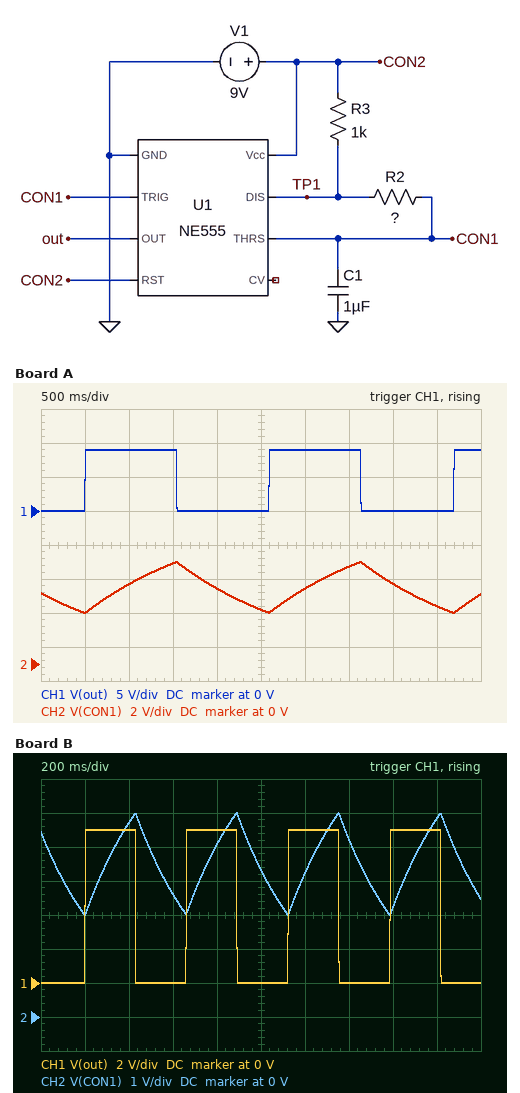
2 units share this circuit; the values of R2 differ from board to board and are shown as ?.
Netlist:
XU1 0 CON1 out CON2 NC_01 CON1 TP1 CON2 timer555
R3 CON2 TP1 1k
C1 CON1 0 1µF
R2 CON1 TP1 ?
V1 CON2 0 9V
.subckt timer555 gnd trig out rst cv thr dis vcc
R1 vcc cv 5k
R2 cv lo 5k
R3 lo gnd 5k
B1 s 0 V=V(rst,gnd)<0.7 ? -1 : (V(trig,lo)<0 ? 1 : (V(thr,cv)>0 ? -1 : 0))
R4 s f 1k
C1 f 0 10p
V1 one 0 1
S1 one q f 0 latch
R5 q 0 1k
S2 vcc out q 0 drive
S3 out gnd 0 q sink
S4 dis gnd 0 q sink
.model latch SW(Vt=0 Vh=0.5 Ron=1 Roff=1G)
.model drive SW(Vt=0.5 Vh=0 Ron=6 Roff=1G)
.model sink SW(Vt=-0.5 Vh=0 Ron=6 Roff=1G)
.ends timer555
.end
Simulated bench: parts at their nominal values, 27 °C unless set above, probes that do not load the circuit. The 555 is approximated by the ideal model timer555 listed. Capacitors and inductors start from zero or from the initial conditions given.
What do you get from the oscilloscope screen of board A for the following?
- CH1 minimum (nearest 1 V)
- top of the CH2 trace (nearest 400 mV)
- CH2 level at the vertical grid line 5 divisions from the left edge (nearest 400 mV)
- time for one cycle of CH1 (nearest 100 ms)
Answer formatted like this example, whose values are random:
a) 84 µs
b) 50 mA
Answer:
a) 0 V
b) 6.0 V
c) 3.2 V
d) 2.1 s
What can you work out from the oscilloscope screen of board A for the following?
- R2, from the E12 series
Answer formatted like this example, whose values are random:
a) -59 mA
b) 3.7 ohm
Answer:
a) 1.5 MΩ
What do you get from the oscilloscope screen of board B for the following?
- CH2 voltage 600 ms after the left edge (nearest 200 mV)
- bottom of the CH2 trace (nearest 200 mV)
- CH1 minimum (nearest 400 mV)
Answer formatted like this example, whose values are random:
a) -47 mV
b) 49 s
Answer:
a) 3.6 V
b) 3.0 V
c) 0 V
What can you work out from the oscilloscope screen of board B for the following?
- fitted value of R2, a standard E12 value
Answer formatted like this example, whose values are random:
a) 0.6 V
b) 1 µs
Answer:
a) 330 kΩ
